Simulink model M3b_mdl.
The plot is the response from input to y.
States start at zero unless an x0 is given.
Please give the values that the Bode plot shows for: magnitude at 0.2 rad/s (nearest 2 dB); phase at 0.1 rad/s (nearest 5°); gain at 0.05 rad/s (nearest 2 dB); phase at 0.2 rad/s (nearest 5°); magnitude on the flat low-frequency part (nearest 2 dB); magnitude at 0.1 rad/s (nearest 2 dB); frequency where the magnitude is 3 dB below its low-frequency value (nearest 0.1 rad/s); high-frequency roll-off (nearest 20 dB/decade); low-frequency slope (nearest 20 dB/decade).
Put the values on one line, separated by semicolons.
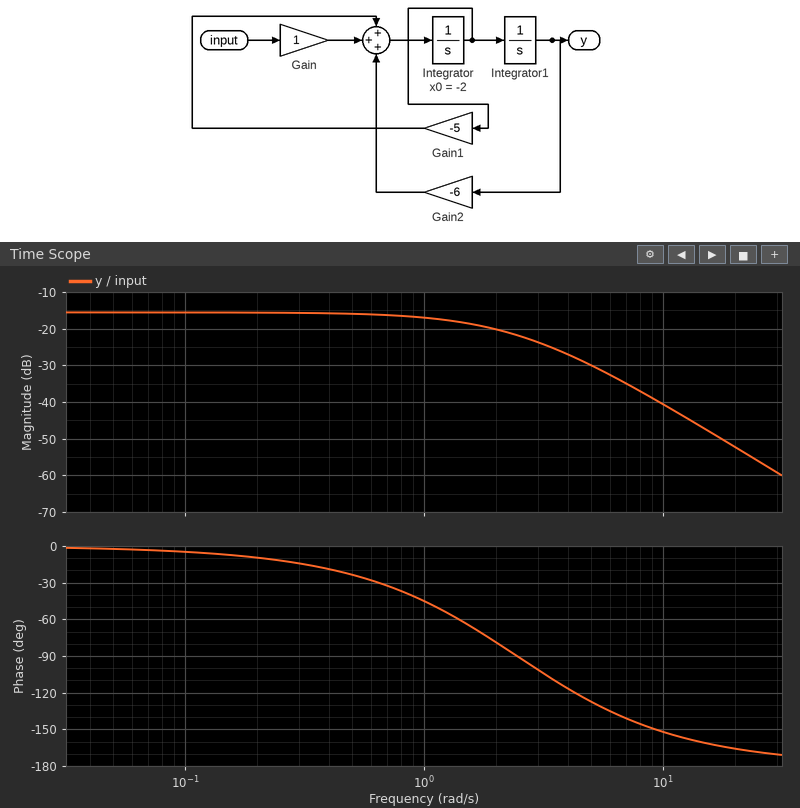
-16 dB; -5°; -16 dB; -10°; -16 dB; -16 dB; 1.5 rad/s; -40 dB/decade; 0 dB/decade
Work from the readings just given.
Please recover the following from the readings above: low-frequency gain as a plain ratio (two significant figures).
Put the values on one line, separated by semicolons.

0.16
